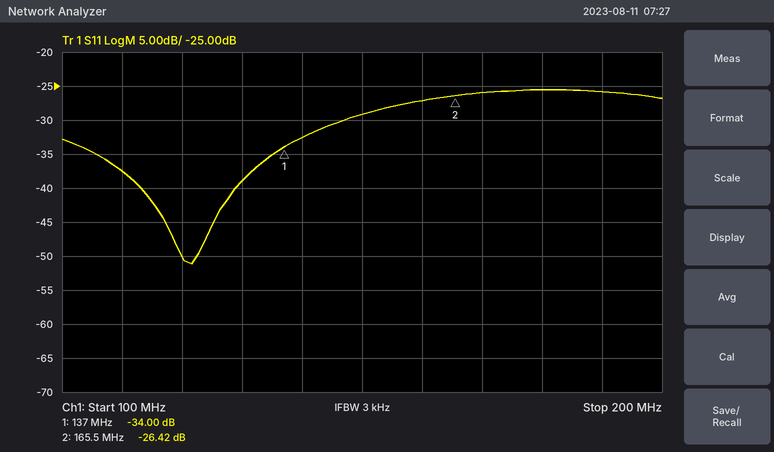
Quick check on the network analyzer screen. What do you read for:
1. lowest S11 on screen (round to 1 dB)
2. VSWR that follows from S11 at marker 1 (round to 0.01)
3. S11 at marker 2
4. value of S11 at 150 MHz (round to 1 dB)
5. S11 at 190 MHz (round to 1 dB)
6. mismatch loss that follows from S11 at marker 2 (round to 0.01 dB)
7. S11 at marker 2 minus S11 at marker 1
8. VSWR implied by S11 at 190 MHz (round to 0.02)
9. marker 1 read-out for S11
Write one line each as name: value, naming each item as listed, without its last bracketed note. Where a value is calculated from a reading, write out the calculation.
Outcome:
lowest S11 on screen: -51 dB
VSWR that follows from S11 at marker 1: (1 + 0.0200)/(1 − 0.0200) ≈ 1.04
S11 at marker 2: -26.42 dB
value of S11 at 150 MHz: -29 dB
S11 at 190 MHz: -26 dB
mismatch loss that follows from S11 at marker 2: −10 log10(1 − 10^(-26.42/10)) ≈ 0.01 dB
S11 at marker 2 minus S11 at marker 1: -26.42 − (-34) = 7.58 dB
VSWR implied by S11 at 190 MHz: |Γ| = 10^(-26/20) = 0.0501; VSWR = (1 + 0.0501)/(1 − 0.0501) ≈ 1.11, so 1.10 to the nearest 0.02
marker 1 read-out for S11: -34.00 dB
